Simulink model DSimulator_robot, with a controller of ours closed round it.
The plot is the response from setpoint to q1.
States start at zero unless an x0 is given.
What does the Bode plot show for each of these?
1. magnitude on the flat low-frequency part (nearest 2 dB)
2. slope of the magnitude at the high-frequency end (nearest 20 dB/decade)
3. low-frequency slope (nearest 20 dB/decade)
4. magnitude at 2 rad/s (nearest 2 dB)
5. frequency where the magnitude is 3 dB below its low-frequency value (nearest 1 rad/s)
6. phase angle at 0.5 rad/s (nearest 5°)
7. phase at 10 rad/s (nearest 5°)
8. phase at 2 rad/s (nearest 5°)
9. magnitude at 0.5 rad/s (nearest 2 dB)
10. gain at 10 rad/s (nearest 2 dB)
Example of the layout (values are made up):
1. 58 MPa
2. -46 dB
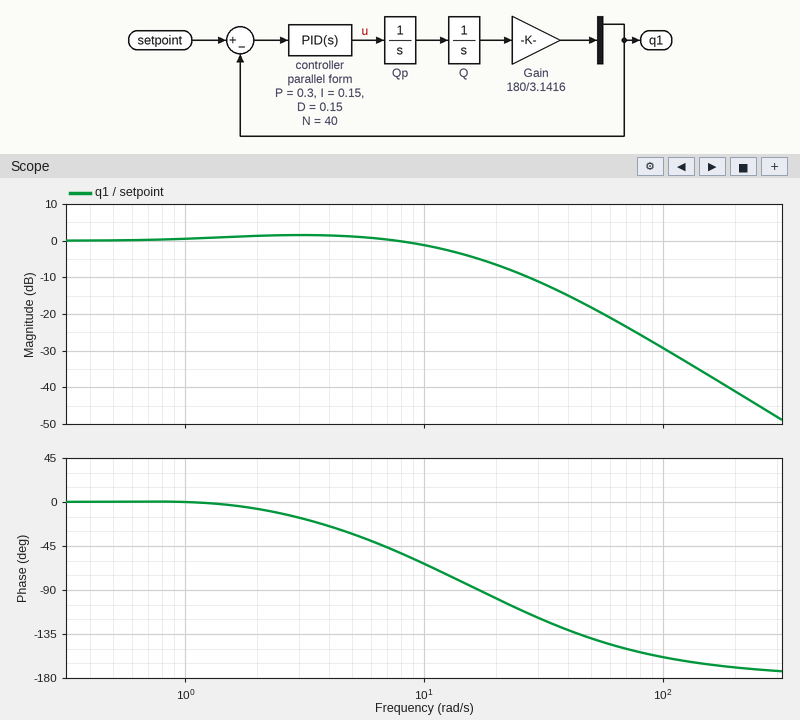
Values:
1. 0 dB
2. -40 dB/decade
3. 0 dB/decade
4. 2 dB
5. 13 rad/s
6. 0°
7. -65°
8. -5°
9. 0 dB
10. -2 dB
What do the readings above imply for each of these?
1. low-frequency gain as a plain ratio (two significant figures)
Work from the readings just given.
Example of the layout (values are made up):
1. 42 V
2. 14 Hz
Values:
1. 1.0
